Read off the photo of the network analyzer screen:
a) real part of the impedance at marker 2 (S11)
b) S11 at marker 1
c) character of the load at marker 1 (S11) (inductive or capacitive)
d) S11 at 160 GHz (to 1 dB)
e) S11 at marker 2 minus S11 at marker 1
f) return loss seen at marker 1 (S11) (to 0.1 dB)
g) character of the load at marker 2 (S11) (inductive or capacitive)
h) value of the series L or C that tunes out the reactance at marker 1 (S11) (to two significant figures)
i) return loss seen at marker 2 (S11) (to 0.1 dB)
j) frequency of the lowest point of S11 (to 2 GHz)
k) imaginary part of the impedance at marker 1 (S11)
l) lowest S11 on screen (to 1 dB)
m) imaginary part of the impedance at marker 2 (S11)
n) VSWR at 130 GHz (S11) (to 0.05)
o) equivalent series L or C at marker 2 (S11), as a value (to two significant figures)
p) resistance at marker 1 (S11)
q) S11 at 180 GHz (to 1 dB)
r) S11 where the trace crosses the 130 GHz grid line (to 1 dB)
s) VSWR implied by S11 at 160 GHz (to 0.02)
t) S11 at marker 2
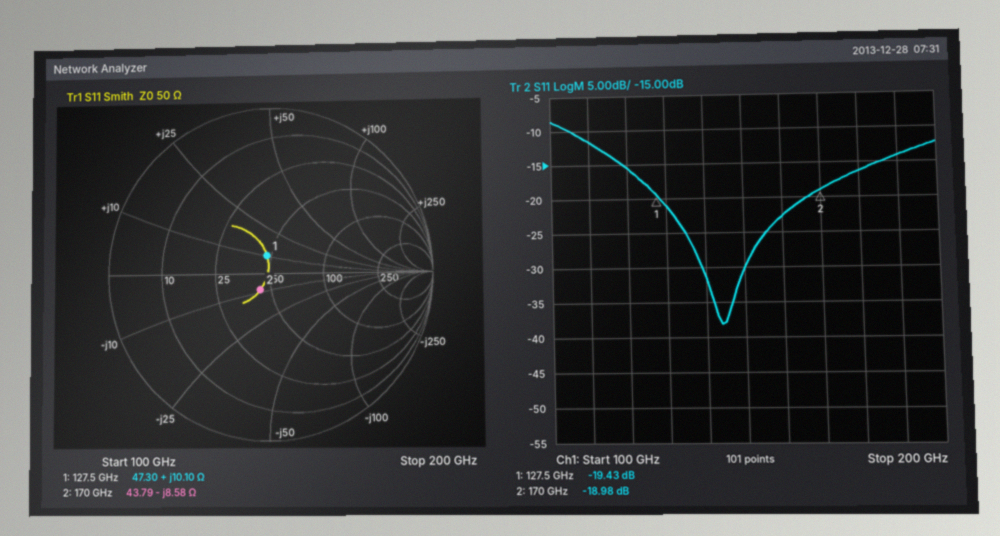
43.79 Ω
-19.43 dB
inductive
-23 dB
0.45 dB
19.4 dB
capacitive
120 fF
19.0 dB
144 GHz
+10.10 Ω
-38 dB
-8.58 Ω
1.20
110 fF
47.30 Ω
-16 dB
-21 dB
1.16
-18.98 dB
